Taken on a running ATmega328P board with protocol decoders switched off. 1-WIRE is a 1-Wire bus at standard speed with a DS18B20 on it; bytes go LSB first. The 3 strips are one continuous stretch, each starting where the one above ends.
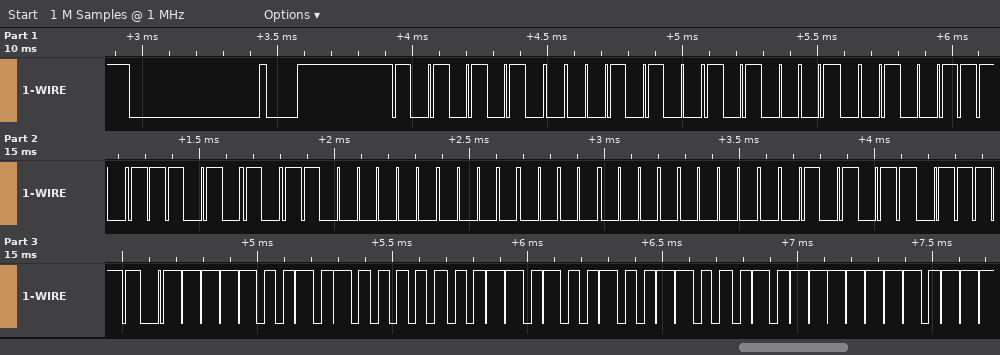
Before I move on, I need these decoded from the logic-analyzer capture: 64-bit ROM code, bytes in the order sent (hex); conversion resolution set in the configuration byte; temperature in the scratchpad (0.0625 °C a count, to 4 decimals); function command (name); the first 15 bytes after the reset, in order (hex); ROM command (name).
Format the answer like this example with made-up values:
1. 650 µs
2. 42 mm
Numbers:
1. 28 45 72 57 03 00 00 D4
2. 12 bits
3. 20.9375 °C
4. Read Scratchpad
5. 55 28 45 72 57 03 00 00 D4 BE 4F 01 4B 46 7F
6. Match ROM
